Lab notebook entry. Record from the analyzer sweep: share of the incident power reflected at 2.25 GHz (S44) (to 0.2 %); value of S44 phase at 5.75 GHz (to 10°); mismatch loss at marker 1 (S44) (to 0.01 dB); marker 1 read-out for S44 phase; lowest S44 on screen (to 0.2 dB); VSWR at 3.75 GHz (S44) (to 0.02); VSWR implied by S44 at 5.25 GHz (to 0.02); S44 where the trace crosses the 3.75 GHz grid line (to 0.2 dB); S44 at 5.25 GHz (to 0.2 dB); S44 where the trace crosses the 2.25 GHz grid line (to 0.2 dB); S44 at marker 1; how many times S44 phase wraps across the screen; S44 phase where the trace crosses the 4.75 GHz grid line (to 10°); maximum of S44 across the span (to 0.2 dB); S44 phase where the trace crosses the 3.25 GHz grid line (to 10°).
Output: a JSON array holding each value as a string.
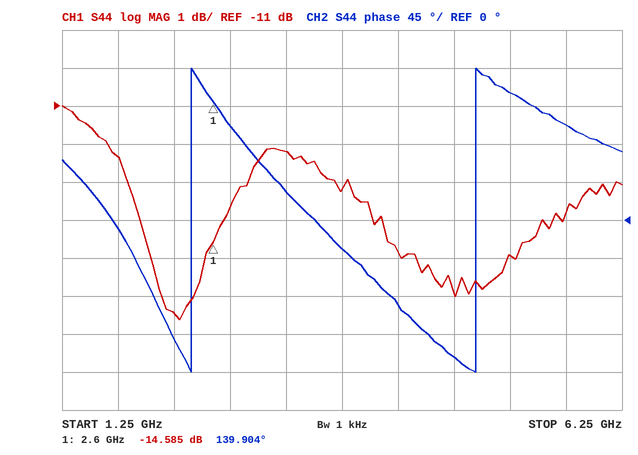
["2.2 %", "110°", "0.15 dB", "139.904°", "-16.6 dB", "1.56", "1.44", "-13.2 dB", "-15.0 dB", "-16.4 dB", "-14.585 dB", "2", "-160°", "-11.0 dB", "30°"]
